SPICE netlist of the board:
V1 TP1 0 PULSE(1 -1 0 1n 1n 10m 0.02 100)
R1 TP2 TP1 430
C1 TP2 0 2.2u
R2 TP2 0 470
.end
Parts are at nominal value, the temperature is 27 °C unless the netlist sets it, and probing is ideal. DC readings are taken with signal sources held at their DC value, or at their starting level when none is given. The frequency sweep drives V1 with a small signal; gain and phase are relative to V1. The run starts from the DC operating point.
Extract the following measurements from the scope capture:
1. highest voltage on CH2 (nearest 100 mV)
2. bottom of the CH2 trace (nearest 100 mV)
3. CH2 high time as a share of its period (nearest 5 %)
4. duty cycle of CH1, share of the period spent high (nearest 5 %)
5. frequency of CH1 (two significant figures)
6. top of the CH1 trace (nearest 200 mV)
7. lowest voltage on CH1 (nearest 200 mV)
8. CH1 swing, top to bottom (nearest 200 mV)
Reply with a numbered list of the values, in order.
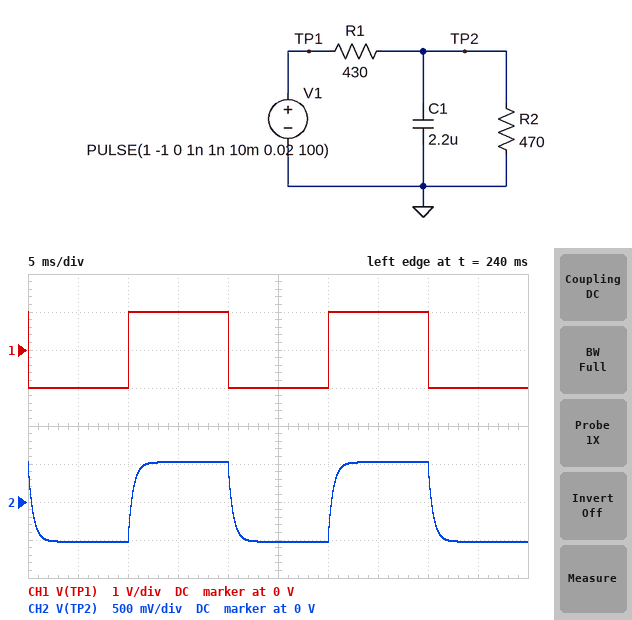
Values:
1. 500 mV
2. -500 mV
3. 50 %
4. 50 %
5. 50 Hz
6. 1.0 V
7. -1.0 V
8. 2.0 V
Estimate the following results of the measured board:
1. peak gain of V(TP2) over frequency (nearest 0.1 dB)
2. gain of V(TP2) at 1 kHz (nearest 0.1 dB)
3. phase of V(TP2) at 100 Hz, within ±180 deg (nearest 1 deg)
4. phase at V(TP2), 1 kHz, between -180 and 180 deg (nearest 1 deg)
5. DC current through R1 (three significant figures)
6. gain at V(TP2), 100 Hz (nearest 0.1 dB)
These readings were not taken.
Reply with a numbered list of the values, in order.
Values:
1. -5.6 dB
2. -15.9 dB
3. -17 deg
4. -72 deg
5. 1.11 mA
6. -6.0 dB
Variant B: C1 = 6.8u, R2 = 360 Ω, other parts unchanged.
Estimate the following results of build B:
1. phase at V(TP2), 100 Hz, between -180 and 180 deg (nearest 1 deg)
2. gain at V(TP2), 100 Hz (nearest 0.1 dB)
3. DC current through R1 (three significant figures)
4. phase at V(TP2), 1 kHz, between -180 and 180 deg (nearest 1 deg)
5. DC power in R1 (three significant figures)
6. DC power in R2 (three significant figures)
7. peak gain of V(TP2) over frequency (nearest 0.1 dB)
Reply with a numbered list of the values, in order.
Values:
1. -40 deg
2. -9.1 dB
3. 1.27 mA
4. -83 deg
5. 689 µW
6. 577 µW
7. -6.8 dB
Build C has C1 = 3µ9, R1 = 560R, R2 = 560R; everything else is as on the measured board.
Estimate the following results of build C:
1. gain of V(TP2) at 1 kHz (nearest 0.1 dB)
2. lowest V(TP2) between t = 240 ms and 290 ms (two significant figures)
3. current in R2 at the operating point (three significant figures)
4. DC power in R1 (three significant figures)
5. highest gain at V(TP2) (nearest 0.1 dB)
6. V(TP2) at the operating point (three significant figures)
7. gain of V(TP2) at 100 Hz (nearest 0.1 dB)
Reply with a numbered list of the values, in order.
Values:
1. -22.8 dB
2. -500 mV
3. 893 µA
4. 446 µW
5. -6.0 dB
6. 500 mV
7. -7.7 dB
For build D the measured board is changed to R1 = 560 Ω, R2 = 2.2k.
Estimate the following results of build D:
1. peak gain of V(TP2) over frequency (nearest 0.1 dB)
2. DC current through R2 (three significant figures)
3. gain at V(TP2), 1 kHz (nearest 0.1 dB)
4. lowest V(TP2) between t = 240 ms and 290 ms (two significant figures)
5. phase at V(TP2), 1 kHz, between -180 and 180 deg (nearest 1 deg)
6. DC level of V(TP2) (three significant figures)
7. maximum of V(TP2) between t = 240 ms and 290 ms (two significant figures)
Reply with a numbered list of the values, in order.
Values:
1. -2.0 dB
2. 362 µA
3. -17.9 dB
4. -800 mV
5. -81 deg
6. 797 mV
7. 800 mV
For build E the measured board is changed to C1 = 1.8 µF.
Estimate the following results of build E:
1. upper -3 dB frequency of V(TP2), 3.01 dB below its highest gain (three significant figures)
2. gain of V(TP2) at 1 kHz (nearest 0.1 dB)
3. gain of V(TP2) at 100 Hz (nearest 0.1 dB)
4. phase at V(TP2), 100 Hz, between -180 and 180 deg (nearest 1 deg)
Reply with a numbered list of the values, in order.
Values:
1. 394 Hz
2. -14.4 dB
3. -5.9 dB
4. -14 deg
